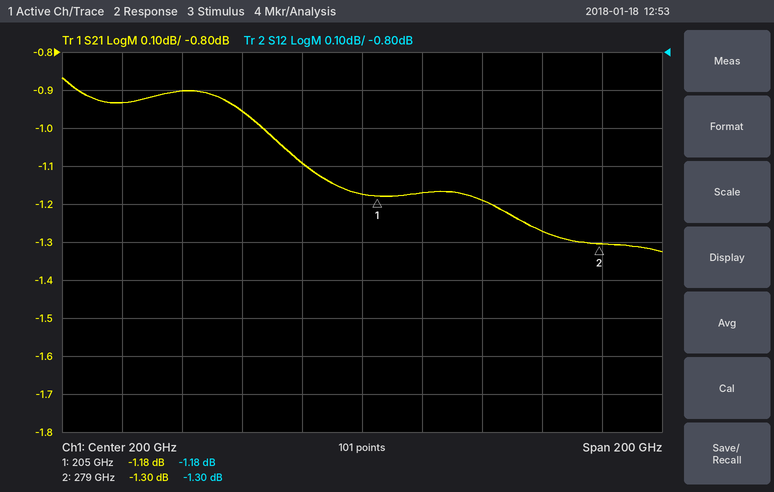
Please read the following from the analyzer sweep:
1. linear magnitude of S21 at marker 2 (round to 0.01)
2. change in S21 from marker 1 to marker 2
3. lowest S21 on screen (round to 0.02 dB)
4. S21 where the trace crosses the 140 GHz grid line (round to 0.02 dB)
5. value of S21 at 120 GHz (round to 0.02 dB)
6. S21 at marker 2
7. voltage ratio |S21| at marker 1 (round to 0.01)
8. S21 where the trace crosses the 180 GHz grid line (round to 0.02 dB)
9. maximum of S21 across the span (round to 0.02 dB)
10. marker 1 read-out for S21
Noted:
0.86
-0.12 dB
-1.32 dB
-0.90 dB
-0.94 dB
-1.30 dB
0.87
-1.10 dB
-0.86 dB
-1.18 dB
